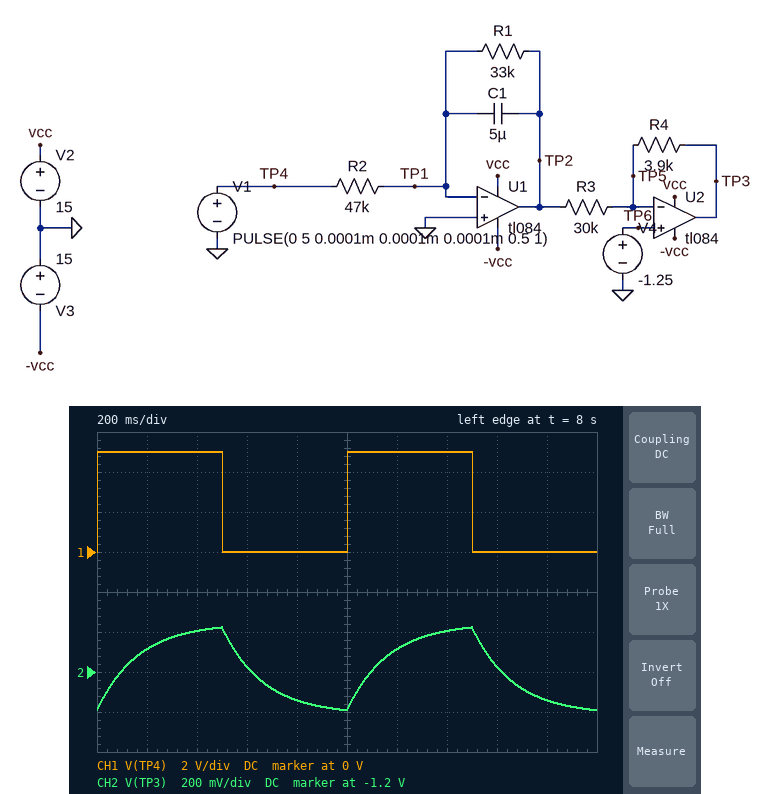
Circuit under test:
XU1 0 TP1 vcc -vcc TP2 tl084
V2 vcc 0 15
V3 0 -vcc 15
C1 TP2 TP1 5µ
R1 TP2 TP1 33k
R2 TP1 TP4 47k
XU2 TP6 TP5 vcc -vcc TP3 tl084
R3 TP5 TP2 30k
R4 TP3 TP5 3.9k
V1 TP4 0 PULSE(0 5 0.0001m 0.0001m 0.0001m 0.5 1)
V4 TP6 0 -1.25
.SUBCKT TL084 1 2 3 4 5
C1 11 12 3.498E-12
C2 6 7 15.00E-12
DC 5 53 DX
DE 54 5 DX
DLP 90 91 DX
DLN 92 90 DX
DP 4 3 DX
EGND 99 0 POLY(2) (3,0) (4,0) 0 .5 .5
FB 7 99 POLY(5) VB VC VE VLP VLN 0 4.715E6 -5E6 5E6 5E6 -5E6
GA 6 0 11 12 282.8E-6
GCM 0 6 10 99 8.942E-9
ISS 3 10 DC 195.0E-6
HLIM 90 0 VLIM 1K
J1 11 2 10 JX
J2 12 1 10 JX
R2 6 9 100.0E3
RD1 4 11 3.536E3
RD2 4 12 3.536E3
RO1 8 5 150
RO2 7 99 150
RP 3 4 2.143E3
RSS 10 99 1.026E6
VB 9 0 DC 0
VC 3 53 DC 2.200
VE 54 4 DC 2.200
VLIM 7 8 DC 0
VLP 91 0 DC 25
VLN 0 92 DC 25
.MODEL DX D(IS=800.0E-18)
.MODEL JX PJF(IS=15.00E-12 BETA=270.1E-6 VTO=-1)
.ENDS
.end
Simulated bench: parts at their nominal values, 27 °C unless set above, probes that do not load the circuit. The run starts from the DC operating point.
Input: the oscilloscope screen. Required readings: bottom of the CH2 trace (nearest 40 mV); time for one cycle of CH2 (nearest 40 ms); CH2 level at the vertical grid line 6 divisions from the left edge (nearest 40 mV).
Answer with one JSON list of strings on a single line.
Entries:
["-1.40 V", "1.00 s", "-1.08 V"]
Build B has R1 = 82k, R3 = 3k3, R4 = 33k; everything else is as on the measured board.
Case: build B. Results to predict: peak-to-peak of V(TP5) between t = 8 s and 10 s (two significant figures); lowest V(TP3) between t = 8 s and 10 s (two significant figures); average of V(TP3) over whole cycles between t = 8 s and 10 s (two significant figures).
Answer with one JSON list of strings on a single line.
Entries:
["3.7 V", "6.1 V", "13 V"]
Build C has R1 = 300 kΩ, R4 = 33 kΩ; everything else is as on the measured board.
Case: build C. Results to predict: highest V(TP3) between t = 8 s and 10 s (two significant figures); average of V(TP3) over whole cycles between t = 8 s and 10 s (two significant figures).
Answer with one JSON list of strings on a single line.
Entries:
["12 V", "11 V"]
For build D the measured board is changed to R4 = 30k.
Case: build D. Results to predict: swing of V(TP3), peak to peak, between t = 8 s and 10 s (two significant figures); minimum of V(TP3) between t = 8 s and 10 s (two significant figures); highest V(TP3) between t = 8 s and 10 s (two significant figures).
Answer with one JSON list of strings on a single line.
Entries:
["3.2 V", "-2.3 V", "850 mV"]
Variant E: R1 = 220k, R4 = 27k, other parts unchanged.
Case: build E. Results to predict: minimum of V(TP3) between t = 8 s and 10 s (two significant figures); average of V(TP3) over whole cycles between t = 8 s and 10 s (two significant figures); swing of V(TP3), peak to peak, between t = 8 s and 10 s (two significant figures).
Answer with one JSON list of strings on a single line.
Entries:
["5.6 V", "7.9 V", "4.1 V"]
